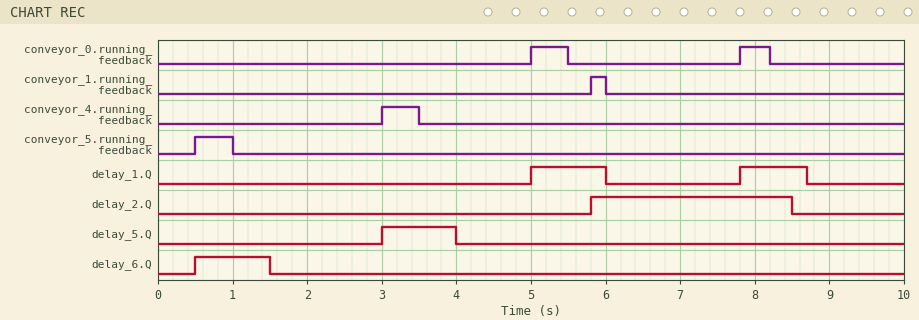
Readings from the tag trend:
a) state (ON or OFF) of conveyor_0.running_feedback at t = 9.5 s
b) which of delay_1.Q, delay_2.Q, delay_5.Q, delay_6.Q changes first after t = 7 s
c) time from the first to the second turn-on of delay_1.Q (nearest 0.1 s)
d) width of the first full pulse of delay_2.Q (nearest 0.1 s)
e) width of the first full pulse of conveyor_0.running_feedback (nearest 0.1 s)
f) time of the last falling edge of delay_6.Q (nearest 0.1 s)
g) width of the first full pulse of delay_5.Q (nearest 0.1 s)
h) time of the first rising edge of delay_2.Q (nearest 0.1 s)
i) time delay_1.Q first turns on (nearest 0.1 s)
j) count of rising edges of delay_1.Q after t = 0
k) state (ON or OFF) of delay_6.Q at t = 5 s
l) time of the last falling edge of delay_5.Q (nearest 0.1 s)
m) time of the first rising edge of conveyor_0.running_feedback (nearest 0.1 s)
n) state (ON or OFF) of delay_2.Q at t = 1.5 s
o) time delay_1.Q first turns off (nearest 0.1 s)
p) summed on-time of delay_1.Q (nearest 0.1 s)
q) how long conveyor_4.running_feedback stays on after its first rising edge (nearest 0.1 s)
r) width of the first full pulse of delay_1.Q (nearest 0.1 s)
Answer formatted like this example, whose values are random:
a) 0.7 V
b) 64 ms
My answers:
a) OFF
b) delay_1.Q
c) 2.8 s
d) 2.7 s
e) 0.5 s
f) 1.5 s
g) 1.0 s
h) 5.8 s
i) 5.0 s
j) 2
k) OFF
l) 4.0 s
m) 5.0 s
n) OFF
o) 6.0 s
p) 1.9 s
q) 0.5 s
r) 1.0 s
